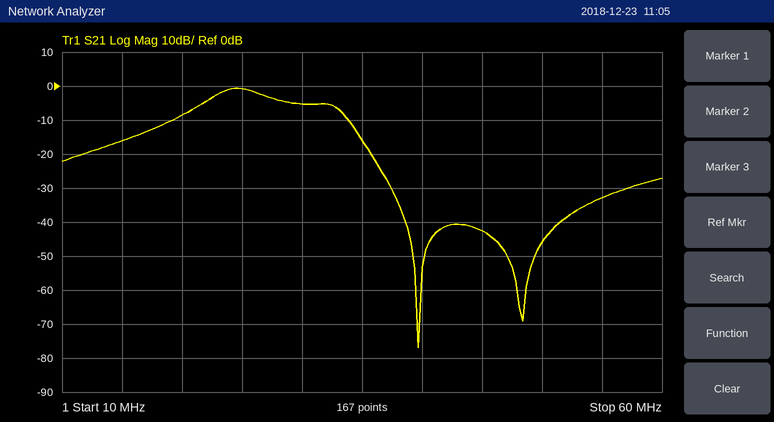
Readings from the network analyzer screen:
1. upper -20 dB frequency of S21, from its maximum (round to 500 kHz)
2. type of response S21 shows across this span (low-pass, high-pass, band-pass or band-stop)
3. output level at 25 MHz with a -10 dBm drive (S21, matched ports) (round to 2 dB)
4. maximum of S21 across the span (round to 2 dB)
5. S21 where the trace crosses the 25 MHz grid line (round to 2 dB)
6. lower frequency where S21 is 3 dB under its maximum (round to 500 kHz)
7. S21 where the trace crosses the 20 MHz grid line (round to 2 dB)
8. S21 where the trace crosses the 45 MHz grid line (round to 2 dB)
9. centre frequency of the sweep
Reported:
36.0 MHz
band-pass
-10 dBm
0 dB
0 dB
22.5 MHz
-8 dB
-42 dB
35 MHz
